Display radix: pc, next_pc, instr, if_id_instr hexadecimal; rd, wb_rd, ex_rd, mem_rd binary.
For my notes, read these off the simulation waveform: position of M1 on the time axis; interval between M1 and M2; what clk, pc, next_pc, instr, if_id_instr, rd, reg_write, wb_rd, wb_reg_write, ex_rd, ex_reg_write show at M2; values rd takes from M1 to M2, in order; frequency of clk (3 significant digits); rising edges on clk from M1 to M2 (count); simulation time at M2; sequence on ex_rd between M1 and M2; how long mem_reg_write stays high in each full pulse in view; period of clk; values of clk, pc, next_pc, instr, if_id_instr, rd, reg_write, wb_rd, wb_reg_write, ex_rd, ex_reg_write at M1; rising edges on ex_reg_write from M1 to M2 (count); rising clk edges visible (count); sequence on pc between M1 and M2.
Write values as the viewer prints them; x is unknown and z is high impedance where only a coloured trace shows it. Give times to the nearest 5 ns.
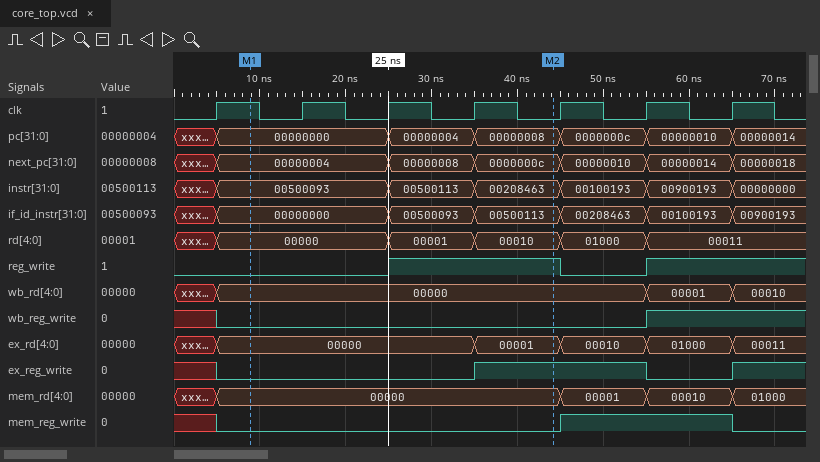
10 ns
35 ns
clk=0, pc=00000008, next_pc=0000000c, instr=00208463, if_id_instr=00500113, rd=00010, reg_write=1, wb_rd=00000, wb_reg_write=0, ex_rd=00001, ex_reg_write=1
00000, 00001, 00010
100 MHz
3
45 ns
00000, 00001
20 ns
10 ns
clk=1, pc=00000000, next_pc=00000004, instr=00500093, if_id_instr=00000000, rd=00000, reg_write=0, wb_rd=00000, wb_reg_write=0, ex_rd=00000, ex_reg_write=0
1
7
00000000, 00000004, 00000008
